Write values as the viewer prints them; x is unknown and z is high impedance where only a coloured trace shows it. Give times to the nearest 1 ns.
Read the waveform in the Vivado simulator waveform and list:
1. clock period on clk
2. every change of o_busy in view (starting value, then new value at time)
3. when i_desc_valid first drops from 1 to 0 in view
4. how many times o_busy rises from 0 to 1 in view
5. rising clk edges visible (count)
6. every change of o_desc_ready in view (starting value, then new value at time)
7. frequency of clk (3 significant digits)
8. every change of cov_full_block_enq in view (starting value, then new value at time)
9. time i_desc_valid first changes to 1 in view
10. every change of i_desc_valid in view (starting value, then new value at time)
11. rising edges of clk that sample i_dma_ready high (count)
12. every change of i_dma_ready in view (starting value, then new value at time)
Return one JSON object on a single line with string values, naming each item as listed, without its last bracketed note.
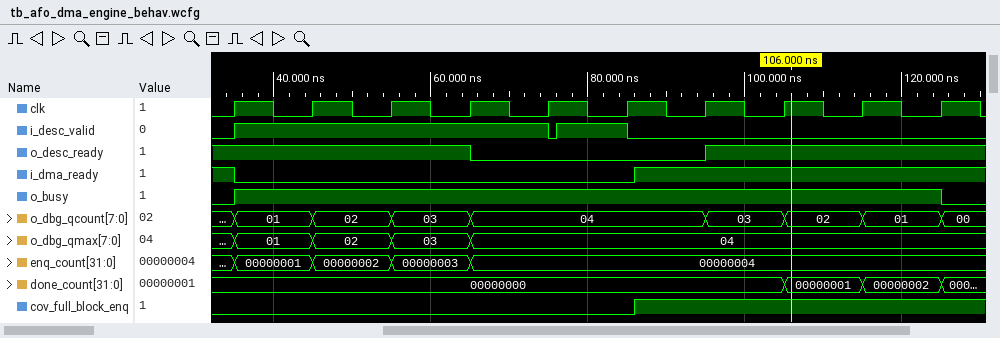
{"clock period on clk": "10 ns", "every change of o_busy in view": "0, 1 at 35 ns, 0 at 125 ns", "when i_desc_valid first drops from 1 to 0 in view": "75 ns", "how many times o_busy rises from 0 to 1 in view": "1", "rising clk edges visible": "10", "every change of o_desc_ready in view": "1, 0 at 65 ns, 1 at 95 ns", "frequency of clk": "100 MHz", "every change of cov_full_block_enq in view": "0, 1 at 86 ns", "time i_desc_valid first changes to 1 in view": "35 ns", "every change of i_desc_valid in view": "0, 1 at 35 ns, 0 at 75 ns, 1 at 76 ns, 0 at 85 ns", "rising edges of clk that sample i_dma_ready high": "5", "every change of i_dma_ready in view": "1, 0 at 35 ns, 1 at 86 ns"}
